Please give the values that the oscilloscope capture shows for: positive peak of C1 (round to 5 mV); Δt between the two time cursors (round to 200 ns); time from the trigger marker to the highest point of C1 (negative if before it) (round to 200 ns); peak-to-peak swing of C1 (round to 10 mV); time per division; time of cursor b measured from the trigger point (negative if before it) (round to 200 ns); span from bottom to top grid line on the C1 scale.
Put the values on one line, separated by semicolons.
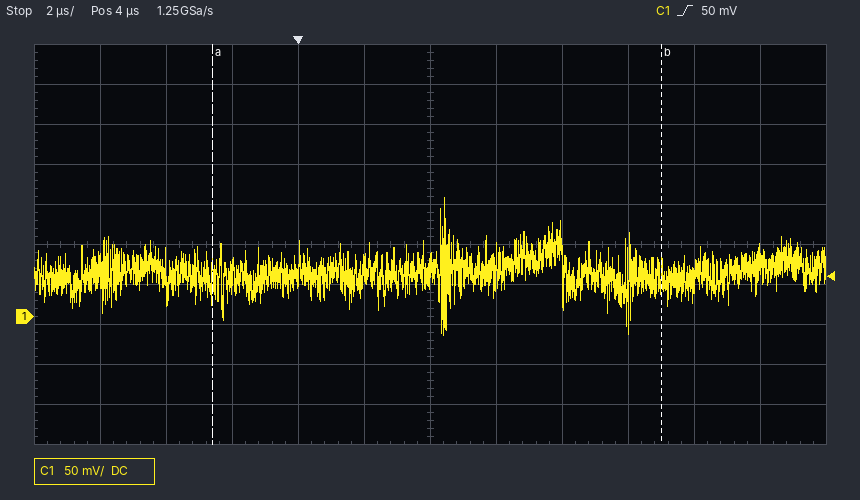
150 mV; 13.6 µs; +4.4 µs; 170 mV; 2 µs; +11.0 µs; 500 mV
